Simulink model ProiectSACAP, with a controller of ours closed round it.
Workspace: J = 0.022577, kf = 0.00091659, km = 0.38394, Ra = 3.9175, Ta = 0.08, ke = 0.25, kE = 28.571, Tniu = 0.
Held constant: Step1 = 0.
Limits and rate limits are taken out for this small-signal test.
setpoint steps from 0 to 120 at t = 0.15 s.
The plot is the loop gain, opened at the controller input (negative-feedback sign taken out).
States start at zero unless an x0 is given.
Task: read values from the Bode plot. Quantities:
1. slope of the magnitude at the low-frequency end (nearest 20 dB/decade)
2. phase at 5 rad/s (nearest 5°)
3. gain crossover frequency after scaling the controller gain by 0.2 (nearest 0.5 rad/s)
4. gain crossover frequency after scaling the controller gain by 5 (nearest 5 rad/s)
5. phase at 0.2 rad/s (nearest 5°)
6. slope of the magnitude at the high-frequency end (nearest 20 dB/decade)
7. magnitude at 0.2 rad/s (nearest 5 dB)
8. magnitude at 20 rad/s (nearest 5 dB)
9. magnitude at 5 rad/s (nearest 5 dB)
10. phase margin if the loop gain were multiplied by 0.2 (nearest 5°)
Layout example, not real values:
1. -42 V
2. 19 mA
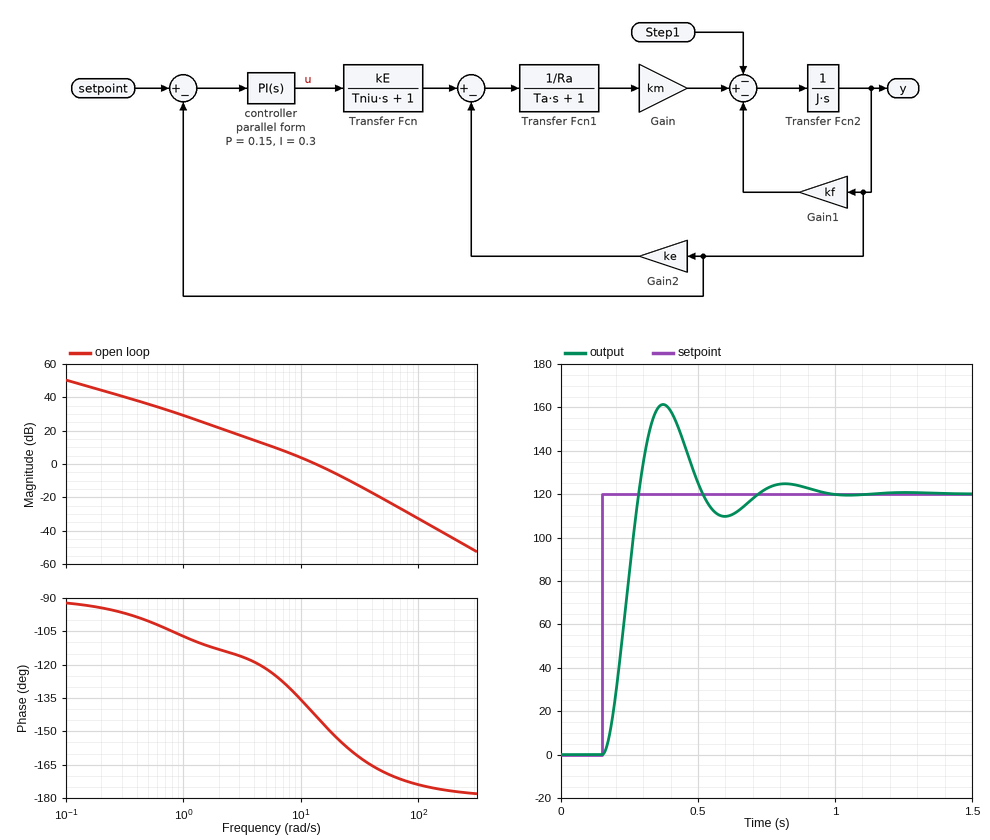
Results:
1. -20 dB/decade
2. -120°
3. 4.0 rad/s
4. 35 rad/s
5. -95°
6. -40 dB/decade
7. 45 dB
8. -5 dB
9. 10 dB
10. 60°
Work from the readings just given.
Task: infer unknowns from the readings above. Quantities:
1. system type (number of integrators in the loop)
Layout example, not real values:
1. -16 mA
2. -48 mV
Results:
1. 1
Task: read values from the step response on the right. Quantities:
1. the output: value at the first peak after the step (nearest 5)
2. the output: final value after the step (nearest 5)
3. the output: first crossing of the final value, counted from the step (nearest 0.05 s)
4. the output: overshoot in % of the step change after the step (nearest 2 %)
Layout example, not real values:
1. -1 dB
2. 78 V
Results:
1. 160
2. 120
3. 0.15 s
4. 34 %
